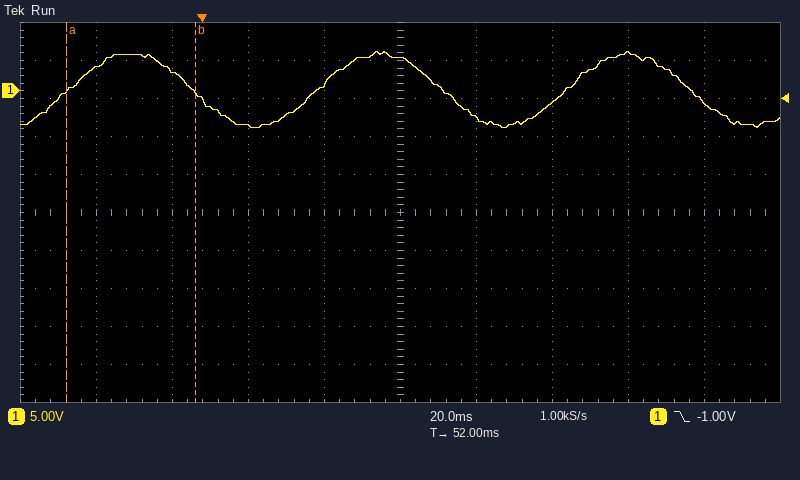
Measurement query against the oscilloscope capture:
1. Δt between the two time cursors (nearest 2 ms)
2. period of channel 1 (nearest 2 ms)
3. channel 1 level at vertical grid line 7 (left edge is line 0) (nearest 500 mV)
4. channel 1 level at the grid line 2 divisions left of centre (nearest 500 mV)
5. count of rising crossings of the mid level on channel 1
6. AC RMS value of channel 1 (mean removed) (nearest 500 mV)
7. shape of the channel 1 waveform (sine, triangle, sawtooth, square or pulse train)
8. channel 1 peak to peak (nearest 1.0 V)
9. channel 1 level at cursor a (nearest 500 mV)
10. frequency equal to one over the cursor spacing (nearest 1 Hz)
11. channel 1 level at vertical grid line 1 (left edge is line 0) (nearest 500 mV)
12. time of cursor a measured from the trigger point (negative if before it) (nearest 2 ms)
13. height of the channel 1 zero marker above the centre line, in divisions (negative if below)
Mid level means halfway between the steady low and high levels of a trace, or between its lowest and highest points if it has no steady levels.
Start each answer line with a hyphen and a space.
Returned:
- 34 ms
- 66 ms
- -1.5 V
- -4.5 V
- 3
- 3.5 V
- sine
- 10.0 V
- 0.0 V
- 29 Hz
- 3.0 V
- -36 ms
- +3.2 div
